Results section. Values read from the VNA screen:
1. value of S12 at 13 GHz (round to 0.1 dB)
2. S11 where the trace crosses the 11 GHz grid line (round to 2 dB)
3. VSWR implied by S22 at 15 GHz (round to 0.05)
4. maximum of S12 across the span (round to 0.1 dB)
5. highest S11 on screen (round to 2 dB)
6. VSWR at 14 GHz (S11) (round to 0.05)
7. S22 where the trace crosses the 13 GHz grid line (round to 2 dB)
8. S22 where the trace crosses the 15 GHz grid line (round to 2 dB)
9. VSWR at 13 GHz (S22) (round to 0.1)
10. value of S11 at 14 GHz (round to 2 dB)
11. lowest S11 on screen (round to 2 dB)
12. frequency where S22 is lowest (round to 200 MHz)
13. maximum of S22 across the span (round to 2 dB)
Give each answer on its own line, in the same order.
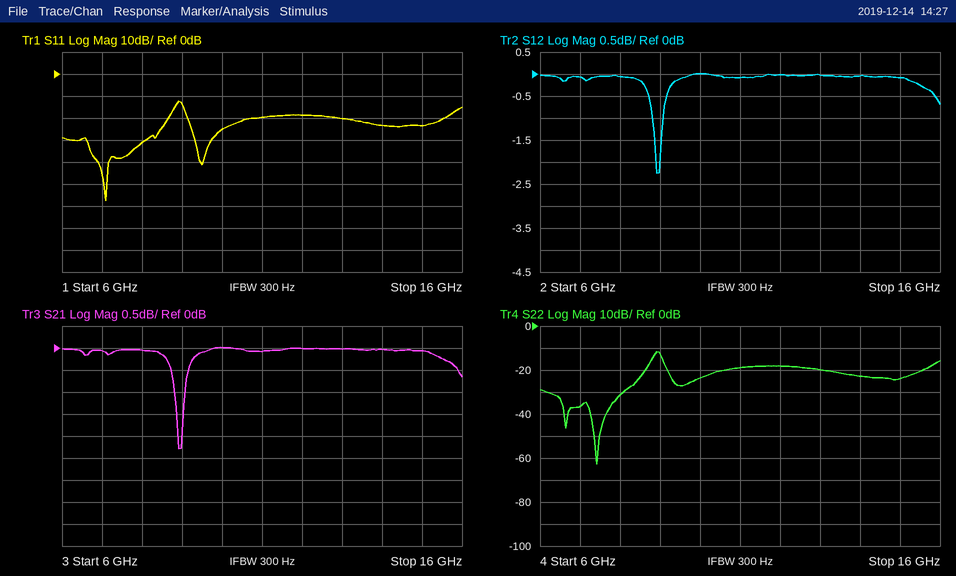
0.0 dB
-20 dB
1.15
0.0 dB
-12 dB
1.15
-20 dB
-24 dB
1.2
-24 dB
-58 dB
7.4 GHz
-12 dB
